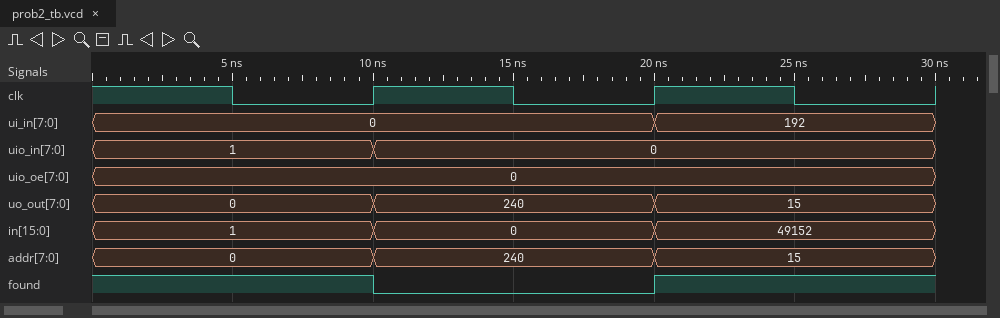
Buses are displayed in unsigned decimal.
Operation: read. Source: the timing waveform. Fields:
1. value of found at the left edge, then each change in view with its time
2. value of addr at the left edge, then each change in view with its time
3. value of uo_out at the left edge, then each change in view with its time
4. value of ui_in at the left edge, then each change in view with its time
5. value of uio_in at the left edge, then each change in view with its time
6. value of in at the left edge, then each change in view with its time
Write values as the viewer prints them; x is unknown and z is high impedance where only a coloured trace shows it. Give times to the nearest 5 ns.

1, 0 at 10 ns, 1 at 20 ns
0, 240 at 10 ns, 15 at 20 ns
0, 240 at 10 ns, 15 at 20 ns
0, 192 at 20 ns
1, 0 at 10 ns
1, 0 at 10 ns, 49152 at 20 ns
